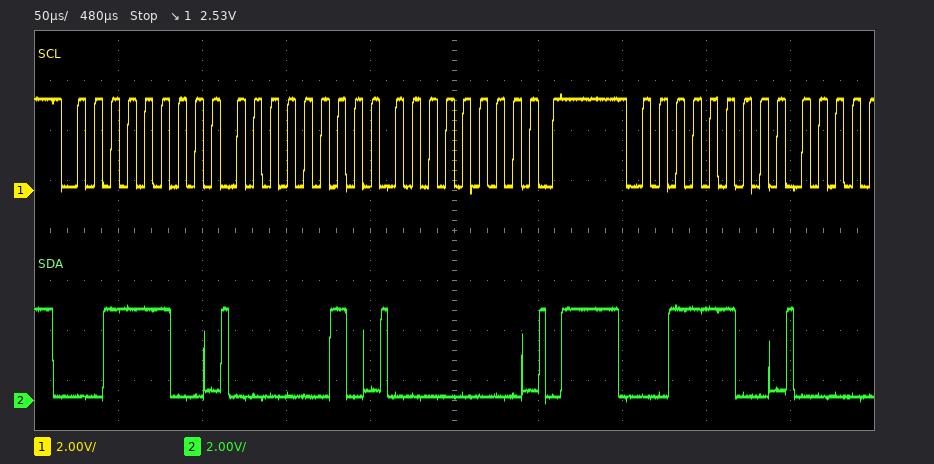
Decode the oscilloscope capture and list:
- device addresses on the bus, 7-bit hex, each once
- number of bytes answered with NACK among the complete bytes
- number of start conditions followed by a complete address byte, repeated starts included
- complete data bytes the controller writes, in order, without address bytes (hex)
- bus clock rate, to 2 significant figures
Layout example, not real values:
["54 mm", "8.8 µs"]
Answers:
["0x1E", "0", "2", "02 00", "100 kHz"]
